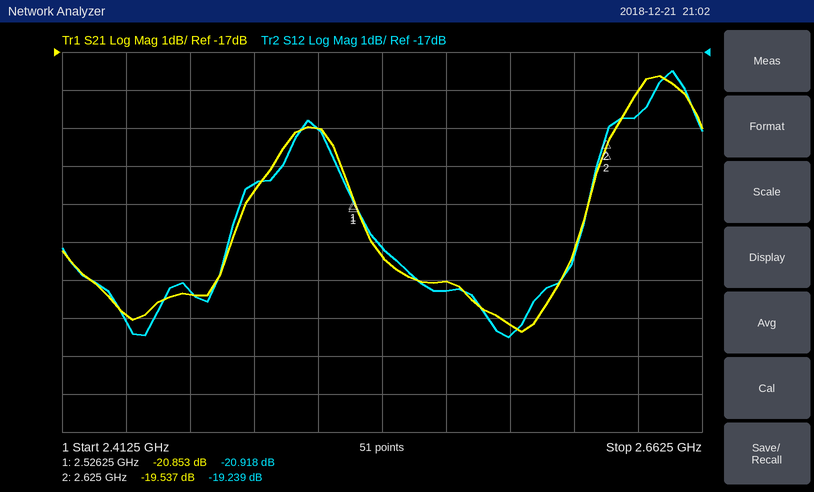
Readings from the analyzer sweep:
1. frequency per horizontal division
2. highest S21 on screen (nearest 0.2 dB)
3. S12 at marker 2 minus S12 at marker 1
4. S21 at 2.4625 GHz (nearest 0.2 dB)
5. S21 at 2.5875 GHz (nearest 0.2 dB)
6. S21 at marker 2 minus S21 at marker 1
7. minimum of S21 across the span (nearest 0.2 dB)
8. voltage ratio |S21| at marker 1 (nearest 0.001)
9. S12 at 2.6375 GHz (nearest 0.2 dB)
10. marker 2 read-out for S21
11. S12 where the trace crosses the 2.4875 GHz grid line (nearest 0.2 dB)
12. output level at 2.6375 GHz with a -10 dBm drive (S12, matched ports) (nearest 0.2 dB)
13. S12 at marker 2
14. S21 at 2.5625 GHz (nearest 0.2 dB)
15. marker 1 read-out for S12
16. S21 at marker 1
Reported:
25 MHz
-17.6 dB
1.679 dB
-23.4 dB
-24.2 dB
1.316 dB
-24.4 dB
0.091
-18.6 dB
-19.537 dB
-20.4 dB
-28.6 dBm
-19.239 dB
-23.0 dB
-20.918 dB
-20.853 dB
